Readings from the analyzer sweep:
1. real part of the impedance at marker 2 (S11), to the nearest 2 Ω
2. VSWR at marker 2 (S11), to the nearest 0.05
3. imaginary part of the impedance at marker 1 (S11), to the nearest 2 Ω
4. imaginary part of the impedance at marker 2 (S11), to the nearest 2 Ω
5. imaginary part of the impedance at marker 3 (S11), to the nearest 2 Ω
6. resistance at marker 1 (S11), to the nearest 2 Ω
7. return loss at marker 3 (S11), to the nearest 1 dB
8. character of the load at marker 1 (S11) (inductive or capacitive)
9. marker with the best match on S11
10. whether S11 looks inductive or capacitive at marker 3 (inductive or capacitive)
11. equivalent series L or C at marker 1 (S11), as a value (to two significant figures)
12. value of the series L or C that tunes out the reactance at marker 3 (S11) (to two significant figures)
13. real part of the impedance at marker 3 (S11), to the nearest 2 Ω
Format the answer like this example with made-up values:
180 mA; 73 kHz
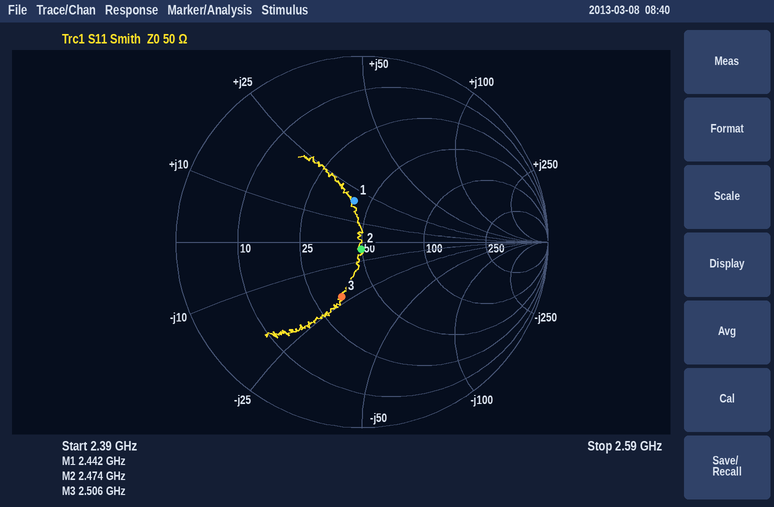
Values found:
50 Ω; 1.10; +20 Ω; -4 Ω; -22 Ω; 42 Ω; 10 dB; inductive; marker 2; capacitive; 1.3 nH; 1.4 nH; 34 Ω
